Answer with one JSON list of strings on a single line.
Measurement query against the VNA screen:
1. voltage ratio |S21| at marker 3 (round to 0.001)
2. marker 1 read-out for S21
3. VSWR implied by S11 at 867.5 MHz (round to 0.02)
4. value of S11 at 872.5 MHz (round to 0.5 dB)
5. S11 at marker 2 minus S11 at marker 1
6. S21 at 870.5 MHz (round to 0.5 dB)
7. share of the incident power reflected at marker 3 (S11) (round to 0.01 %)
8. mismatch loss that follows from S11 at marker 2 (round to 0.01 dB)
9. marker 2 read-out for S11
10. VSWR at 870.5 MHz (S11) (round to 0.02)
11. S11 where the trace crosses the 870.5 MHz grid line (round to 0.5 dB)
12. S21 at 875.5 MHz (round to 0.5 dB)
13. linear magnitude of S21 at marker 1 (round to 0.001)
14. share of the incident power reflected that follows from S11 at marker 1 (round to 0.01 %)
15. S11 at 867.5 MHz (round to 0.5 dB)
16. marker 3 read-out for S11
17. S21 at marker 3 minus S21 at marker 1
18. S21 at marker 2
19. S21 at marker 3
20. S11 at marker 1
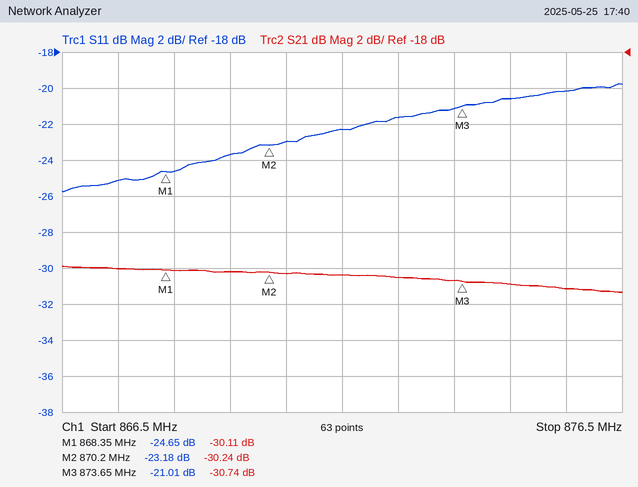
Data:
["0.029", "-30.11 dB", "1.12", "-21.5 dB", "1.47 dB", "-30.5 dB", "0.79 %", "0.02 dB", "-23.18 dB", "1.16", "-23.0 dB", "-31.0 dB", "0.031", "0.34 %", "-25.0 dB", "-21.01 dB", "-0.63 dB", "-30.24 dB", "-30.74 dB", "-24.65 dB"]
